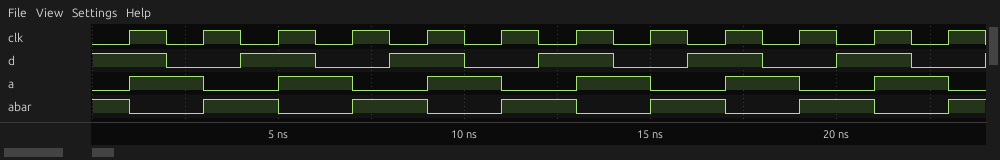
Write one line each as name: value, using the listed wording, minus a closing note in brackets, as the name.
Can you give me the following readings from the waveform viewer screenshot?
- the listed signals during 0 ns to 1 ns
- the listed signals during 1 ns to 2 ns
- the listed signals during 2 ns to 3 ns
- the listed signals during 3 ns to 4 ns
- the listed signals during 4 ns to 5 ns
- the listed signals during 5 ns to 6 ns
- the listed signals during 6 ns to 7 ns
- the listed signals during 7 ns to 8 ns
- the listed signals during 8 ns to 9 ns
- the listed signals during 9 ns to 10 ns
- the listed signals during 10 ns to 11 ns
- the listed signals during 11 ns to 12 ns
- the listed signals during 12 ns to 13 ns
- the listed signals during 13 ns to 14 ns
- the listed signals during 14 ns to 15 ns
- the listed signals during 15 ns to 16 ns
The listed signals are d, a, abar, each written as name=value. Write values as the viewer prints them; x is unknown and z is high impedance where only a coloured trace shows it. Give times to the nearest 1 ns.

the listed signals during 0 ns to 1 ns: d=1, a=0, abar=1
the listed signals during 1 ns to 2 ns: d=1, a=1, abar=0
the listed signals during 2 ns to 3 ns: d=0, a=1, abar=0
the listed signals during 3 ns to 4 ns: d=0, a=0, abar=1
the listed signals during 4 ns to 5 ns: d=1, a=0, abar=1
the listed signals during 5 ns to 6 ns: d=1, a=1, abar=0
the listed signals during 6 ns to 7 ns: d=0, a=1, abar=0
the listed signals during 7 ns to 8 ns: d=0, a=0, abar=1
the listed signals during 8 ns to 9 ns: d=1, a=0, abar=1
the listed signals during 9 ns to 10 ns: d=1, a=1, abar=0
the listed signals during 10 ns to 11 ns: d=0, a=1, abar=0
the listed signals during 11 ns to 12 ns: d=0, a=0, abar=1
the listed signals during 12 ns to 13 ns: d=1, a=0, abar=1
the listed signals during 13 ns to 14 ns: d=1, a=1, abar=0
the listed signals during 14 ns to 15 ns: d=0, a=1, abar=0
the listed signals during 15 ns to 16 ns: d=0, a=0, abar=1
